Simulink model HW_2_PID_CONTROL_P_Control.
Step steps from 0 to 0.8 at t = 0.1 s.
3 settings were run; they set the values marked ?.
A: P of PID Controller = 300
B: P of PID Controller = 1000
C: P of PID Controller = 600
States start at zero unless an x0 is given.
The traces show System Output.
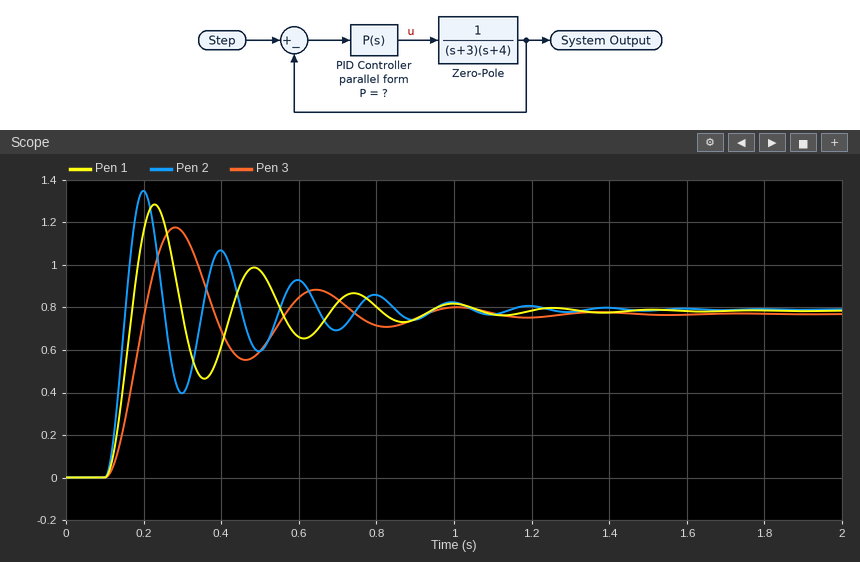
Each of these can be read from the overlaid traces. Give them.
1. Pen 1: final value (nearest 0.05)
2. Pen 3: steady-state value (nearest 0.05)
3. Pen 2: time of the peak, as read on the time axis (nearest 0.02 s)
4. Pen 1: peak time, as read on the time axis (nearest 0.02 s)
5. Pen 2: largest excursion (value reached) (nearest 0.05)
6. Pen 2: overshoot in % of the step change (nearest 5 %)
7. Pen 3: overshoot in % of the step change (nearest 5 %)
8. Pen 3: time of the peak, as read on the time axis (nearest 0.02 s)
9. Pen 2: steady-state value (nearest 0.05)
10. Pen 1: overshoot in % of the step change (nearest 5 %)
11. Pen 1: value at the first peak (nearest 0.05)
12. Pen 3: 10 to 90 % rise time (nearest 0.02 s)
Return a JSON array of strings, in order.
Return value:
["0.80", "0.75", "0.20 s", "0.22 s", "1.35", "70 %", "55 %", "0.28 s", "0.80", "65 %", "1.30", "0.06 s"]
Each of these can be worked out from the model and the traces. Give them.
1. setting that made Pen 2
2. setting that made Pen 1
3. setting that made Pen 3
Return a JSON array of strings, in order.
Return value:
["B", "C", "A"]
